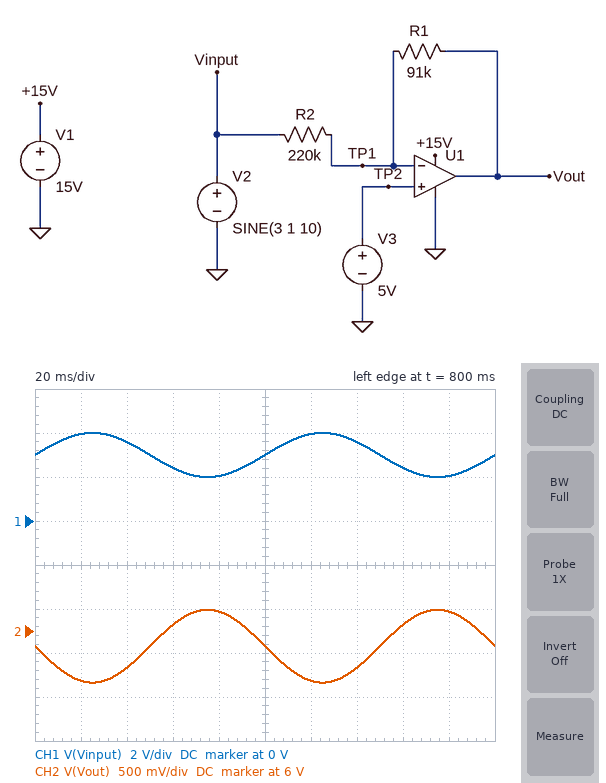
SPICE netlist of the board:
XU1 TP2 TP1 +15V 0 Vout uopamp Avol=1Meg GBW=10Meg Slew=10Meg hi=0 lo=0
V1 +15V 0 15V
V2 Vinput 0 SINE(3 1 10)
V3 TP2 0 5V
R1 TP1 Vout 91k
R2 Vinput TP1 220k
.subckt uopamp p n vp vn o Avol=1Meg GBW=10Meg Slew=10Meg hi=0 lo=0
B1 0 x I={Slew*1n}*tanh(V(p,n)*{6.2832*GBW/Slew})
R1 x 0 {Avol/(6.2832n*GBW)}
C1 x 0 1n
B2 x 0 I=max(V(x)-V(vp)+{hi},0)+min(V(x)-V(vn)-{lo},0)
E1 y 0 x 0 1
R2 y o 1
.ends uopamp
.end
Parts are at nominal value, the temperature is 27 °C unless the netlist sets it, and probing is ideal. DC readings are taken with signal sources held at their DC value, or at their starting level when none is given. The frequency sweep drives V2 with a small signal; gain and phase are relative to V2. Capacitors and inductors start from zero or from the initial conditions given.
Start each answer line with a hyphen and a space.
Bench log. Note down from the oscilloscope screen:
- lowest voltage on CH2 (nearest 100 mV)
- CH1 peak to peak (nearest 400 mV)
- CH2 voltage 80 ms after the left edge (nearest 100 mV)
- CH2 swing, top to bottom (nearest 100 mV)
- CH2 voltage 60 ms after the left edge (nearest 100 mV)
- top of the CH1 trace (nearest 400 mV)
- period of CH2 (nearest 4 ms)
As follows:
- 5.4 V
- 2.0 V
- 6.2 V
- 800 mV
- 6.1 V
- 4.0 V
- 100 ms
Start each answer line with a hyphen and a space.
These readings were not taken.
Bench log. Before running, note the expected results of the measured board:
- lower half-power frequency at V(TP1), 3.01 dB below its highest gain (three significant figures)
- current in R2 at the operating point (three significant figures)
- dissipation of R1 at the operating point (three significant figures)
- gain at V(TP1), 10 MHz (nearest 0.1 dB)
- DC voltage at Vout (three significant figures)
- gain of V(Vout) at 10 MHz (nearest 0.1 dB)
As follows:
- 7.07 MHz
- 9.09 µA
- 7.52 µW
- -12.4 dB
- 5.83 V
- -12.4 dB
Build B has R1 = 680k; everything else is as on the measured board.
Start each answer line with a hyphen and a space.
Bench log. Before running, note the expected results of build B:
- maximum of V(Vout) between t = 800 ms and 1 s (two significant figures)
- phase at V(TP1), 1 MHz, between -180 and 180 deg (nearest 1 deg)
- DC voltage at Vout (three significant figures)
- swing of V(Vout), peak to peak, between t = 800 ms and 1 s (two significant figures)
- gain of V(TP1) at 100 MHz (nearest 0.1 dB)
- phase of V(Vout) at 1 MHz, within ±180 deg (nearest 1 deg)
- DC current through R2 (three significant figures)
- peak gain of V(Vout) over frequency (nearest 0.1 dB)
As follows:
- 14 V
- 68 deg
- 11.2 V
- 6.2 V
- -2.4 dB
- 158 deg
- 9.09 µA
- 9.8 dB
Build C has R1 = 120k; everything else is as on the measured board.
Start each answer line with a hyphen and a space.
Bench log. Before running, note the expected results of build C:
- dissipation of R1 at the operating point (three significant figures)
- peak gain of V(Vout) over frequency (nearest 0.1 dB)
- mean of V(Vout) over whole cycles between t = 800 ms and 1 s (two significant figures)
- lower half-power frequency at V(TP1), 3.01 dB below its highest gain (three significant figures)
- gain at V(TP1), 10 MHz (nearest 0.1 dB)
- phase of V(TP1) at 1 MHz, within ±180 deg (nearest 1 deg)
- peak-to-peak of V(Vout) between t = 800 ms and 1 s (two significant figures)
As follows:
- 9.92 µW
- -5.3 dB
- 6.1 V
- 6.47 MHz
- -10.6 dB
- 81 deg
- 1.1 V
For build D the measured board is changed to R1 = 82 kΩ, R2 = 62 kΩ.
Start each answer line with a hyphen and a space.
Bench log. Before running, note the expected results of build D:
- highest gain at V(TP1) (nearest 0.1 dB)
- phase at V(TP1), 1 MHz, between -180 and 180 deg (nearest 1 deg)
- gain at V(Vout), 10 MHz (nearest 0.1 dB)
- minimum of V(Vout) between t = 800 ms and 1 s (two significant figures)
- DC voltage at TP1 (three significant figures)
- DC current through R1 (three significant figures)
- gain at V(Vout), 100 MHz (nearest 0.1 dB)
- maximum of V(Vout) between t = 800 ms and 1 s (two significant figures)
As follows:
- -4.9 dB
- 77 deg
- -5.6 dB
- 6.3 V
- 5.00 V
- 32.3 µA
- -24.9 dB
- 9.0 V
